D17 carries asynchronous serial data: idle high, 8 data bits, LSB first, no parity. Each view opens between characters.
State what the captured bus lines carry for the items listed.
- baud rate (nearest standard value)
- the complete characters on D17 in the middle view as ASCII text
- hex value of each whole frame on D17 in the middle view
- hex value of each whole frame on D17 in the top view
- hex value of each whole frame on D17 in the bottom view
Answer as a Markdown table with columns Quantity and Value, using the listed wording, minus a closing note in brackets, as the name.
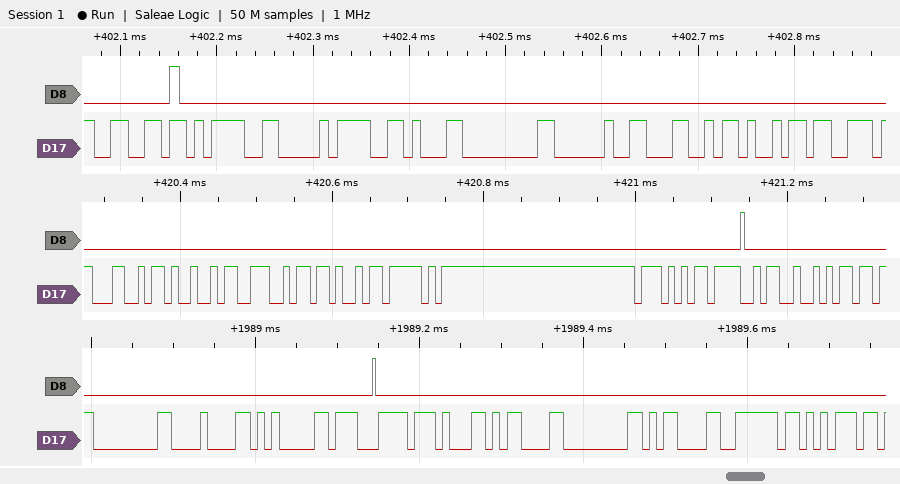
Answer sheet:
| Quantity | Value |
|---|---|
| baud rate | 115200 baud |
| the complete characters on D17 in the middle view as ASCII text | "LINK_WOR" |
| hex value of each whole frame on D17 in the middle view | 4C, 49, 4E, 4B, 5F, 57, 4F, 52 |
| hex value of each whole frame on D17 in the top view | 66, 3D, D0, 16, 00, 20, 4C, 69 |
| hex value of each whole frame on D17 in the bottom view | 00, 08, 05, C7, 17, 0D, 00, 0D, 7E, 75 |
